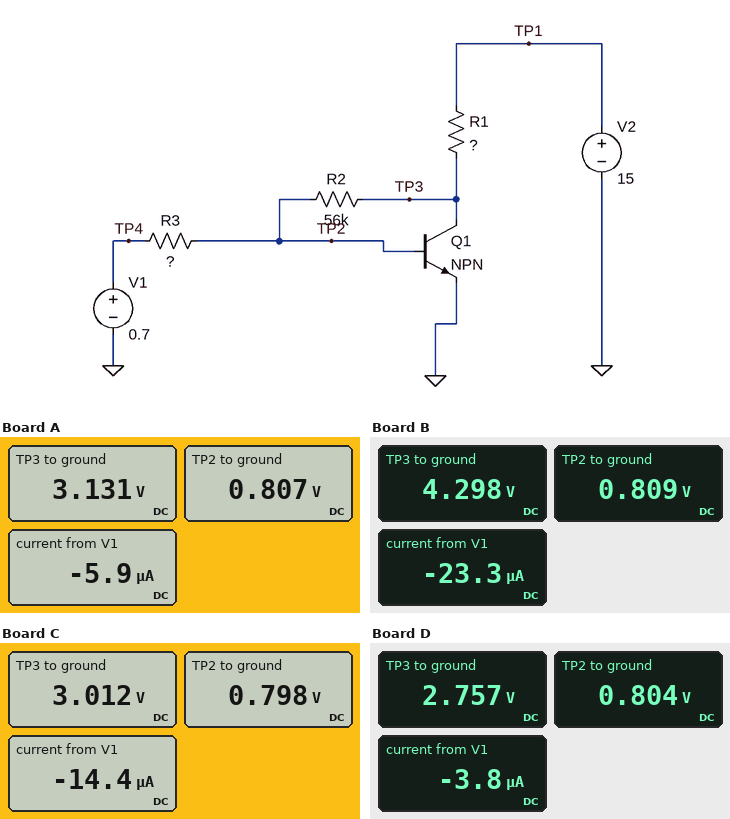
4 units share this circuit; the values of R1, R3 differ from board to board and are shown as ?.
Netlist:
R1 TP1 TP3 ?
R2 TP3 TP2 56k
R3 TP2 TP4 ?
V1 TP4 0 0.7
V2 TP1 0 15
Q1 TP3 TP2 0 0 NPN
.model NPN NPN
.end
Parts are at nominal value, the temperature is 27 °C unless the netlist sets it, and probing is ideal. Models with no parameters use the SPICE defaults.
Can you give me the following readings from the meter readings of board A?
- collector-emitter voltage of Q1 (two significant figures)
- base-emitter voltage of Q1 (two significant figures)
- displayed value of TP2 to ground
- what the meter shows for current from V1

3.1 V
810 mV
0.807 V
-5.9 µA
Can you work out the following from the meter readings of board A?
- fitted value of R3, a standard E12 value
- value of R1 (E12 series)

18 kΩ
3.3 kΩ
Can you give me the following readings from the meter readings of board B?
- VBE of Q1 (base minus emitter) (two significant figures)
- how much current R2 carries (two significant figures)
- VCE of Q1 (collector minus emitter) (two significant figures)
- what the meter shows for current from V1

810 mV
62 µA
4.3 V
-23.3 µA
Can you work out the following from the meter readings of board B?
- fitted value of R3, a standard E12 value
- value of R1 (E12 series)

4.7 kΩ
2.7 kΩ
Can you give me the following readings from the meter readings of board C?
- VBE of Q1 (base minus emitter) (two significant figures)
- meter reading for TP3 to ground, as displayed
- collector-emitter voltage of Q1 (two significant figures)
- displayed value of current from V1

800 mV
3.012 V
3.0 V
-14.4 µA
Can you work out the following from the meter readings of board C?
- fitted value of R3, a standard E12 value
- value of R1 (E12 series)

6.8 kΩ
4.7 kΩ
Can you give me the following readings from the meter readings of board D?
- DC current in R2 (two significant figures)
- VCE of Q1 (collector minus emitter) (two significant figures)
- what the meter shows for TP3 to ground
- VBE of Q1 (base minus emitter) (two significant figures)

35 µA
2.8 V
2.757 V
800 mV
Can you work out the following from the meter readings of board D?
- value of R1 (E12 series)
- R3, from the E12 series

3.9 kΩ
27 kΩ
